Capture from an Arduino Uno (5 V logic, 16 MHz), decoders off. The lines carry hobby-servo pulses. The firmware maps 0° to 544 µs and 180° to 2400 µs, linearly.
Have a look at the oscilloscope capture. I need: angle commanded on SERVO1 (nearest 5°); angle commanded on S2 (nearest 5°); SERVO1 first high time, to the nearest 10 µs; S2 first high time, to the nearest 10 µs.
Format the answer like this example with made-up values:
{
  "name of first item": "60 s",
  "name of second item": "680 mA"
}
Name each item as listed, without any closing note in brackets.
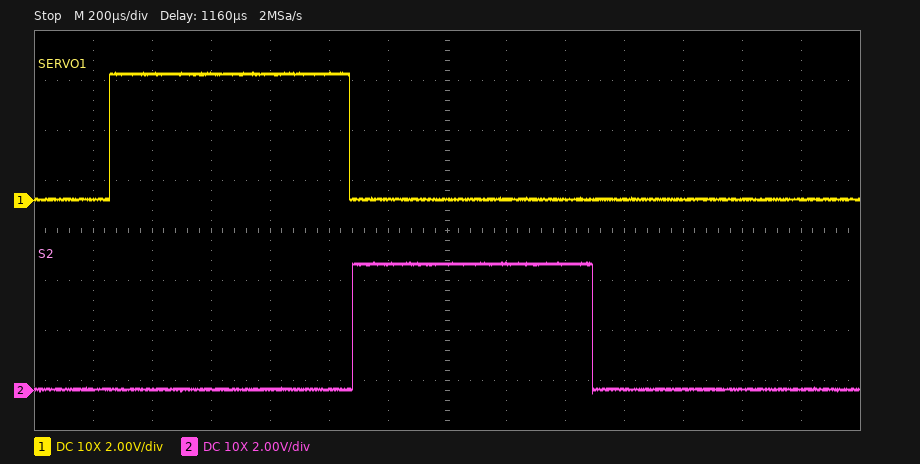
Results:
{
  "angle commanded on SERVO1": "25°",
  "angle commanded on S2": "25°",
  "SERVO1 first high time, to the nearest 10 µs": "810 µs",
  "S2 first high time, to the nearest 10 µs": "810 µs"
}
